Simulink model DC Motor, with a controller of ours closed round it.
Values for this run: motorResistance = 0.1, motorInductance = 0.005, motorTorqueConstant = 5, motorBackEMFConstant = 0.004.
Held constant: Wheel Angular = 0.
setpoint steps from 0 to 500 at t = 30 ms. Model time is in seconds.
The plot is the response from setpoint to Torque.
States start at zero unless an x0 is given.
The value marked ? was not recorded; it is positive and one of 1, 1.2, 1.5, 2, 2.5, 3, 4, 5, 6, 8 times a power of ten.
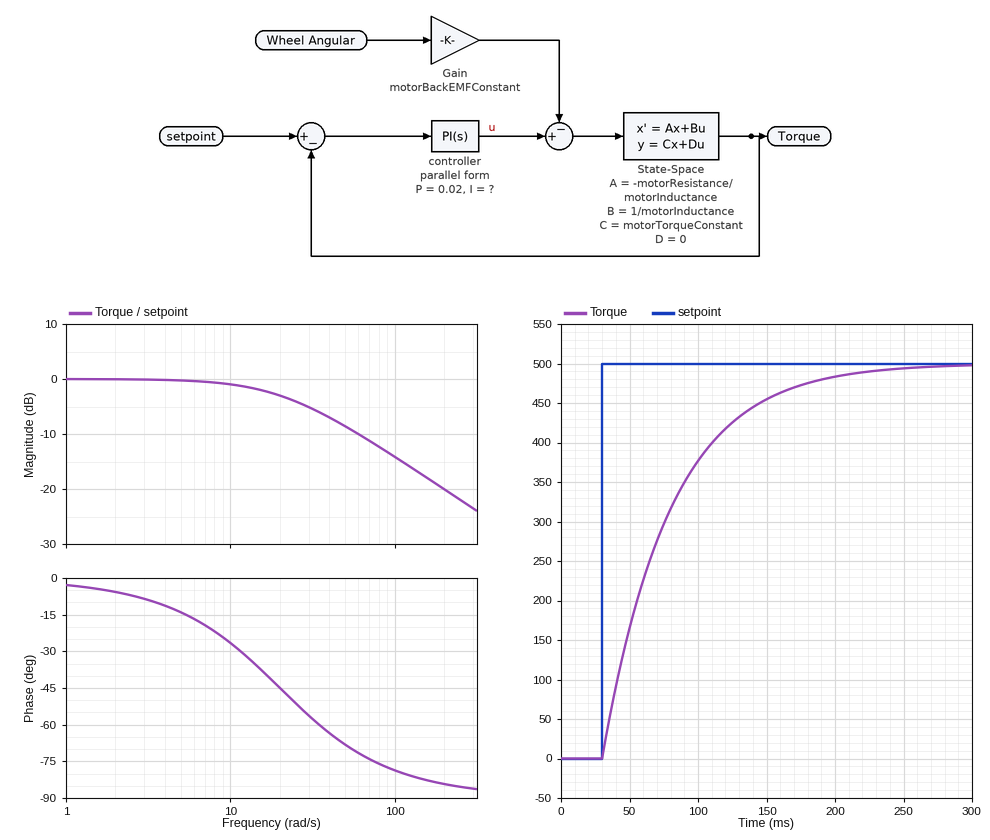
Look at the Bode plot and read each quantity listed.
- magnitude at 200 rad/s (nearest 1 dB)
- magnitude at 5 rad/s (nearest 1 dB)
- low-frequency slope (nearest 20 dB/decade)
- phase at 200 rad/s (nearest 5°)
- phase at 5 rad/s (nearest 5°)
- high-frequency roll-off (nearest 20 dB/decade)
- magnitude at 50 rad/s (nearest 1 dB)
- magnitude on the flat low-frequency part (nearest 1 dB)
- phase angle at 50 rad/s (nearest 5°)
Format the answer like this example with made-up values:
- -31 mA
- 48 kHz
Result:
- -20 dB
- 0 dB
- 0 dB/decade
- -85°
- -15°
- -20 dB/decade
- -9 dB
- 0 dB
- -70°
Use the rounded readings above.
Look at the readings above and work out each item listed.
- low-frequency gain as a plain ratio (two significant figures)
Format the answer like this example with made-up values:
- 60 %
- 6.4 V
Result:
- 1.0
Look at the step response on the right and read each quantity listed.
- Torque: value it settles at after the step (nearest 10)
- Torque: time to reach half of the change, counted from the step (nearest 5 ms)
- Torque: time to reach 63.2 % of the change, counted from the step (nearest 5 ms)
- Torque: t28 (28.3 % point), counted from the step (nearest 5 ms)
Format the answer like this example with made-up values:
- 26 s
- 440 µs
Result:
- 500
- 35 ms
- 50 ms
- 15 ms
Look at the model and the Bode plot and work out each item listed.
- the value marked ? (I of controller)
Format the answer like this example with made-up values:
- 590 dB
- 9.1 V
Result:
- 0.4
